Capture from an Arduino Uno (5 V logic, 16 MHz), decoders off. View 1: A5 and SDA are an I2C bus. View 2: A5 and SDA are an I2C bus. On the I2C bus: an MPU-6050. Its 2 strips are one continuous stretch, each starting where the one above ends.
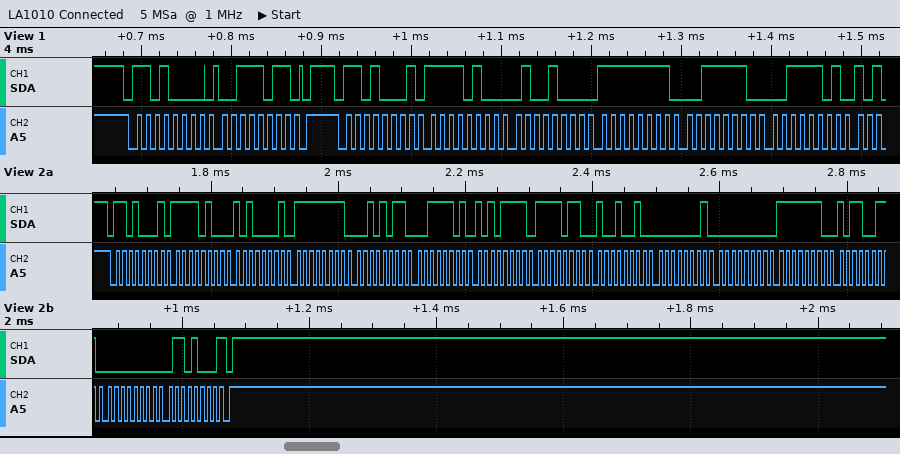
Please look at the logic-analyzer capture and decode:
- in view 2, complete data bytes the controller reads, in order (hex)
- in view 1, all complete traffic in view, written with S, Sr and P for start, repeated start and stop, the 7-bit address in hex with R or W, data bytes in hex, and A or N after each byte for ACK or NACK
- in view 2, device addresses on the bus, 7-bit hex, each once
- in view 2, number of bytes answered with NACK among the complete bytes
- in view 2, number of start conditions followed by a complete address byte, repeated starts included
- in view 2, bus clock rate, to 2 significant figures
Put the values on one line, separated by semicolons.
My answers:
F4 A1 FF 2B 3D AF F6 92 01 00 FE B3 00 68; S 68W A 3B A P S 68R A F4 A 48 A FF A 3E A 3D A; 0x68; 1; 1; 100 kHz
